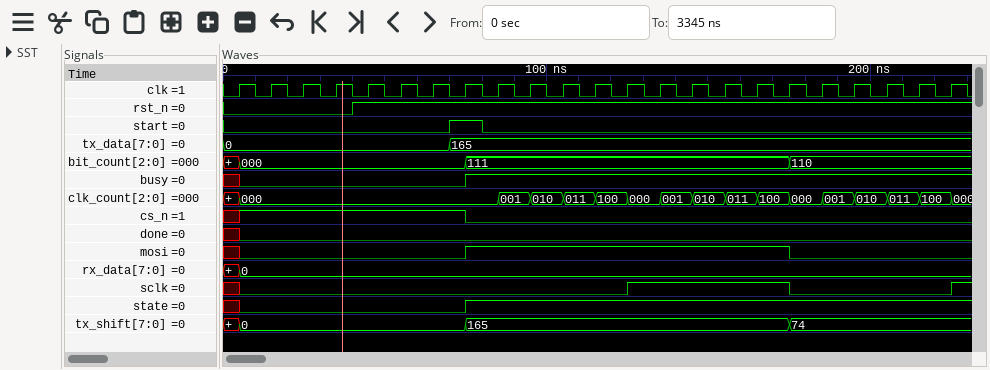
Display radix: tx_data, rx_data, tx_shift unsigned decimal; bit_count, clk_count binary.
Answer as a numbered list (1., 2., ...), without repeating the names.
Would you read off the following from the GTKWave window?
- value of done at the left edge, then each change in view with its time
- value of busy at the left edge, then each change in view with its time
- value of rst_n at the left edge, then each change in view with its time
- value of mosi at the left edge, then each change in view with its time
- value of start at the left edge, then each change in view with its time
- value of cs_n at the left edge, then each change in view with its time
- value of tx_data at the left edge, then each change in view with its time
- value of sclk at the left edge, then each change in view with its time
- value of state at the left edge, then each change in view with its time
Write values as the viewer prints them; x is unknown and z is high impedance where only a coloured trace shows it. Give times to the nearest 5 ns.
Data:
1. x, 0 at 5 ns
2. x, 0 at 5 ns, 1 at 75 ns
3. 0, 1 at 40 ns
4. x, 0 at 5 ns, 1 at 75 ns, 0 at 175 ns
5. 0, 1 at 70 ns, 0 at 80 ns
6. x, 1 at 5 ns, 0 at 75 ns
7. 0, 165 at 70 ns
8. x, 0 at 5 ns, 1 at 125 ns, 0 at 175 ns, 1 at 225 ns
9. x, 0 at 5 ns, 1 at 75 ns
